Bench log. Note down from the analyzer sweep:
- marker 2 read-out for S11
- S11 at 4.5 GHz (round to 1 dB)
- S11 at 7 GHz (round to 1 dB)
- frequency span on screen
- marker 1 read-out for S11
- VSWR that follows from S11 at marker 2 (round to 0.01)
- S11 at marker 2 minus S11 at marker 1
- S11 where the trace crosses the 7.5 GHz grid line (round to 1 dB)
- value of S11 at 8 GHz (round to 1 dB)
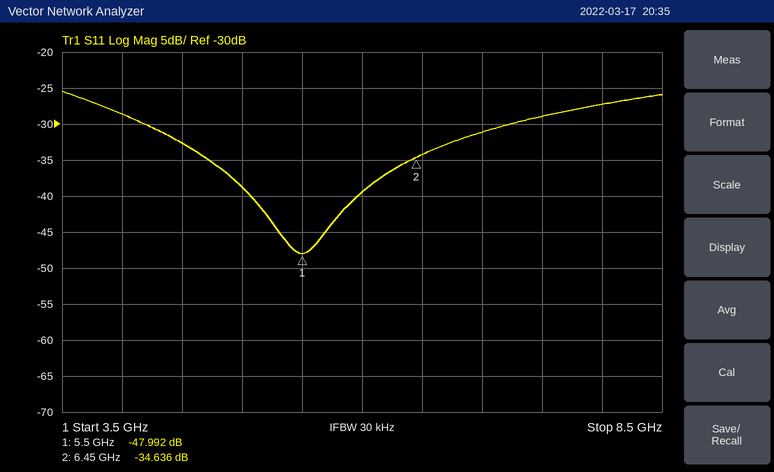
-34.636 dB
-33 dB
-31 dB
5 GHz
-47.992 dB
1.04
13.356 dB
-29 dB
-27 dB
